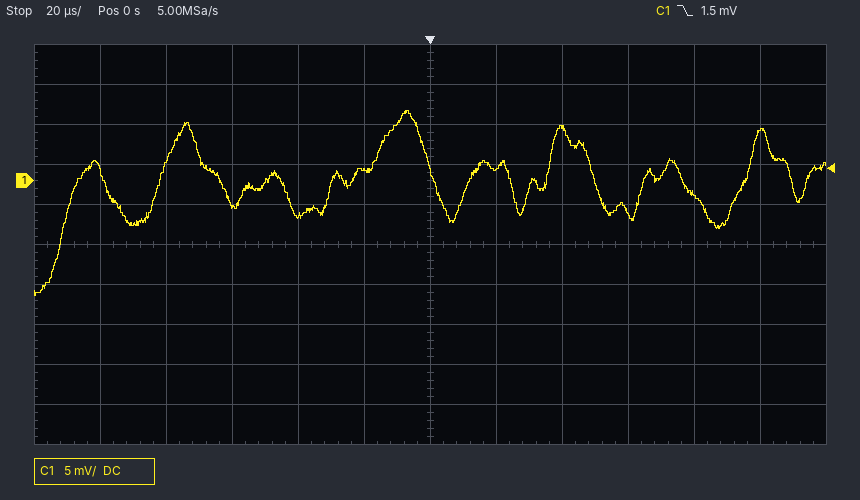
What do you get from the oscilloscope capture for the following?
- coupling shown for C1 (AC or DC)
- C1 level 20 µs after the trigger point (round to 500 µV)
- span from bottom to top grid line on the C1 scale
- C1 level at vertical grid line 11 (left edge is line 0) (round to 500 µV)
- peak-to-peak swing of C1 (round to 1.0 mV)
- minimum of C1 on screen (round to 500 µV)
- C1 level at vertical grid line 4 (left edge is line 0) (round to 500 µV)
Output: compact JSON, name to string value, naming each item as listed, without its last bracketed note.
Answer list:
{"coupling shown for C1": "DC", "C1 level 20 µs after the trigger point": "1.5 mV", "span from bottom to top grid line on the C1 scale": "50 mV", "C1 level at vertical grid line 11 (left edge is line 0)": "6.0 mV", "peak-to-peak swing of C1": "23.0 mV", "minimum of C1 on screen": "-14.5 mV", "C1 level at vertical grid line 4 (left edge is line 0)": "-4.5 mV"}
